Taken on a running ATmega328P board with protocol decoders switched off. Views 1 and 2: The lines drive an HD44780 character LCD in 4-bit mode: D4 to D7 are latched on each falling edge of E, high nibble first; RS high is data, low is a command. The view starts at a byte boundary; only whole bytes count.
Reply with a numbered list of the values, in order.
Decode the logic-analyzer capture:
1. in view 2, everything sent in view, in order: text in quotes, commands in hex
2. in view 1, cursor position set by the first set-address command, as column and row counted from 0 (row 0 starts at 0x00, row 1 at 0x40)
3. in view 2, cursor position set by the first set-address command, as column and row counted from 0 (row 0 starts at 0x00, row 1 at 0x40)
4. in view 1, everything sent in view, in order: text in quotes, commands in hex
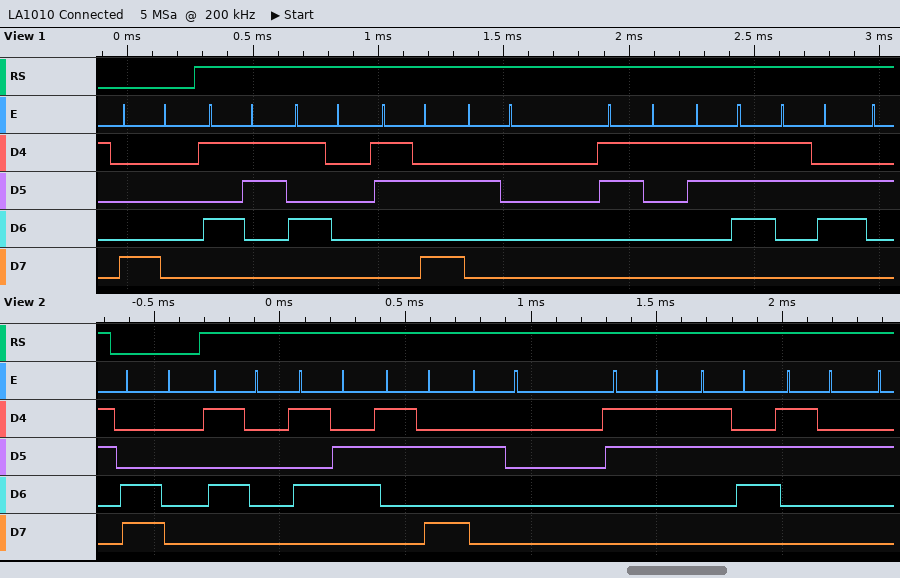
1. 0xC0 "PV: 362"
2. column 0, row 0
3. column 0, row 1
4. 0x80 "SP: 176"
